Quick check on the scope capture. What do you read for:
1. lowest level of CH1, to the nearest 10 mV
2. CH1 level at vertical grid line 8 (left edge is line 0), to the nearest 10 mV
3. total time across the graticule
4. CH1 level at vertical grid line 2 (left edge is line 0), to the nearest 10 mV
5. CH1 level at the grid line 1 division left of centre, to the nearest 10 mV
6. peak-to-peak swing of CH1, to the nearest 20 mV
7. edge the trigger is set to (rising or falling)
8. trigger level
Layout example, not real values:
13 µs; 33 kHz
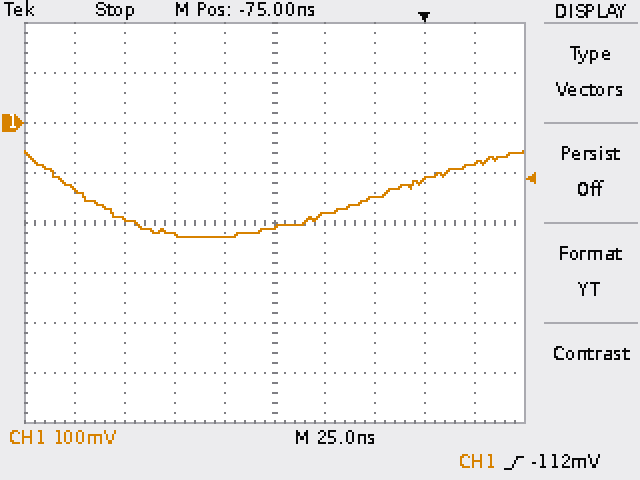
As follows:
-230 mV; -110 mV; 250 ns; -190 mV; -230 mV; 180 mV; rising; -112 mV
